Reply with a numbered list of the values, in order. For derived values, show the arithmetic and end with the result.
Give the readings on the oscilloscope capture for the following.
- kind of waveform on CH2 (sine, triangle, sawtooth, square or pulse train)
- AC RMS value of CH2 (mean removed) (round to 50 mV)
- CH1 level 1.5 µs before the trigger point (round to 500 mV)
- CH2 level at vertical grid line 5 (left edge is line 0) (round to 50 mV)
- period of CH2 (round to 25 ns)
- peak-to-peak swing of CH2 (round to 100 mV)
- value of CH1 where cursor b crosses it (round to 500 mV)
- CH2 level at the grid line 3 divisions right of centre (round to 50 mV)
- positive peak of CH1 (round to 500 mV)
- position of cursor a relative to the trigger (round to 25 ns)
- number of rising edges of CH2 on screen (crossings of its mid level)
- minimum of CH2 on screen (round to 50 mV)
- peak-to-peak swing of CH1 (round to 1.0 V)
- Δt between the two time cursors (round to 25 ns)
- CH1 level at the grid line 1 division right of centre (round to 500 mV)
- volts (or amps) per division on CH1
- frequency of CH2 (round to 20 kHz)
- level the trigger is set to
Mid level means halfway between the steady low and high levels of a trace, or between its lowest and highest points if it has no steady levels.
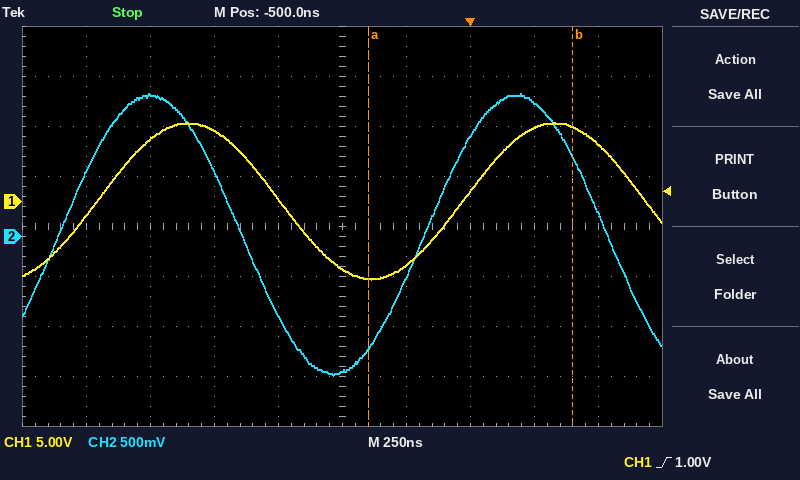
1. sine
2. 2.80 V / (2√2) ≈ 0.990 V, so 1.00 V to the nearest 50 mV
3. -1.5 V
4. -1.35 V
5. 1.425 µs
6. 2.80 V
7. 7.5 V
8. 1.35 V
9. 8.0 V
10. -400 ns
11. 2
12. -1.40 V
13. 16.0 V
14. 800 ns
15. -6.5 V
16. 5 V
17. 1 / 1.425 µs ≈ 702 kHz, so 700 kHz to the nearest 20 kHz
18. 1.00 V
